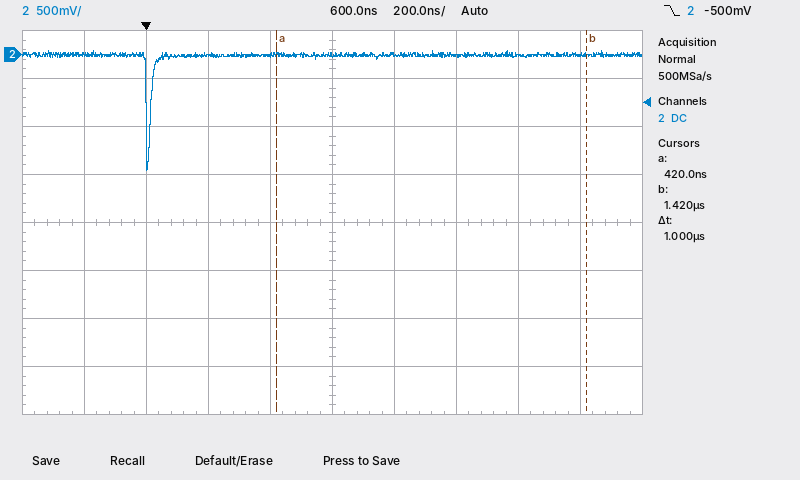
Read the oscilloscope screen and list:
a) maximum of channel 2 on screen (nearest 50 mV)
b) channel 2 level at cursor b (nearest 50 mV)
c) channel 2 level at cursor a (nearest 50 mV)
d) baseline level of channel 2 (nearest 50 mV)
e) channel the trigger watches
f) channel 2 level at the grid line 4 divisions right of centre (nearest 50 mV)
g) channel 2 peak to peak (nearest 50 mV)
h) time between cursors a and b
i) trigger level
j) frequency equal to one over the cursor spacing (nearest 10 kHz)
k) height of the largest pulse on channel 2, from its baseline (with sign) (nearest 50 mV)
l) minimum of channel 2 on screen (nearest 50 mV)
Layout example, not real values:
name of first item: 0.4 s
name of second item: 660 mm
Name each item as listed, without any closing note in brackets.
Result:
maximum of channel 2 on screen: 50 mV
channel 2 level at cursor b: 0 mV
channel 2 level at cursor a: 0 mV
baseline level of channel 2: 0 mV
channel the trigger watches: channel 2
channel 2 level at the grid line 4 divisions right of centre: 0 mV
channel 2 peak to peak: 1.25 V
time between cursors a and b: 1 µs
trigger level: -500 mV
frequency equal to one over the cursor spacing: 1.00 MHz
height of the largest pulse on channel 2, from its baseline (with sign): -1.20 V
minimum of channel 2 on screen: -1.20 V
